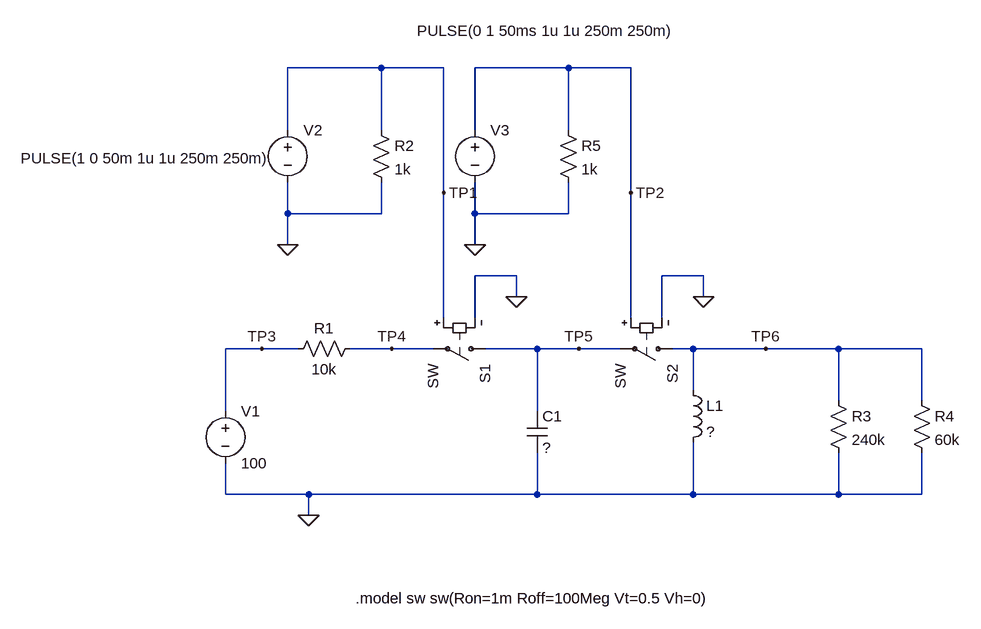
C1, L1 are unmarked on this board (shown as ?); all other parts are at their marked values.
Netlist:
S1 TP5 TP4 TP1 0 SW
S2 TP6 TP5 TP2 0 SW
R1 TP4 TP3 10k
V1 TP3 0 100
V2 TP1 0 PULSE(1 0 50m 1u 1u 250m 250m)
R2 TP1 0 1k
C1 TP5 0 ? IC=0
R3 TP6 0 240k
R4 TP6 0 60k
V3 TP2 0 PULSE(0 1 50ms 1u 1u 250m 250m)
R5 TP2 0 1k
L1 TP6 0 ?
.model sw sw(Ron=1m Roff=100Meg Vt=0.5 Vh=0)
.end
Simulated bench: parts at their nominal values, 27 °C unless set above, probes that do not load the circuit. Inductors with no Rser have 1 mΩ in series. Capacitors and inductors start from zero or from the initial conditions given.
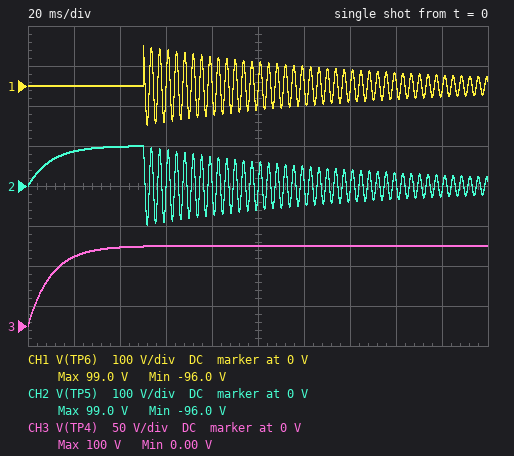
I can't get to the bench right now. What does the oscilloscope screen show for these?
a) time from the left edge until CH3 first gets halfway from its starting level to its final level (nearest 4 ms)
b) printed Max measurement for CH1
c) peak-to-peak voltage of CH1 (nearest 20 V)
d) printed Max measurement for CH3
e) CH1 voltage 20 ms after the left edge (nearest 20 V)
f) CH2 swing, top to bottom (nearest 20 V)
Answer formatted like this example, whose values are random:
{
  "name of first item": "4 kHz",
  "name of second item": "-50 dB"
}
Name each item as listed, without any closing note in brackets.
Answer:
{
  "time from the left edge until CH3 first gets halfway from its starting level to its final level": "8 ms",
  "printed Max measurement for CH1": "99.0 V",
  "peak-to-peak voltage of CH1": "200 V",
  "printed Max measurement for CH3": "100 V",
  "CH1 voltage 20 ms after the left edge": "0 V",
  "CH2 swing, top to bottom": "200 V"
}
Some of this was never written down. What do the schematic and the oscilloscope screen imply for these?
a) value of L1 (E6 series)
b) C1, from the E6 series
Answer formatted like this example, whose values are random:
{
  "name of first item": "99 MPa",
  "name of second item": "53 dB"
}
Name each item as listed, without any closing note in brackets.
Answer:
{
  "value of L1": "330 mH",
  "C1, from the E6 series": "1 µF"
}
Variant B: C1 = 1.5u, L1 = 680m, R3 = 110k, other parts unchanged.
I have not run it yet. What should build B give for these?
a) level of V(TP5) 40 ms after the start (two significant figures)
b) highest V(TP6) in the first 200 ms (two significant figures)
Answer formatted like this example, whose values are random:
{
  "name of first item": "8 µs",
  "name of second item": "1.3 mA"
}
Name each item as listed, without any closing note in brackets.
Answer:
{
  "level of V(TP5) 40 ms after the start": "93 V",
  "highest V(TP6) in the first 200 ms": "96 V"
}
